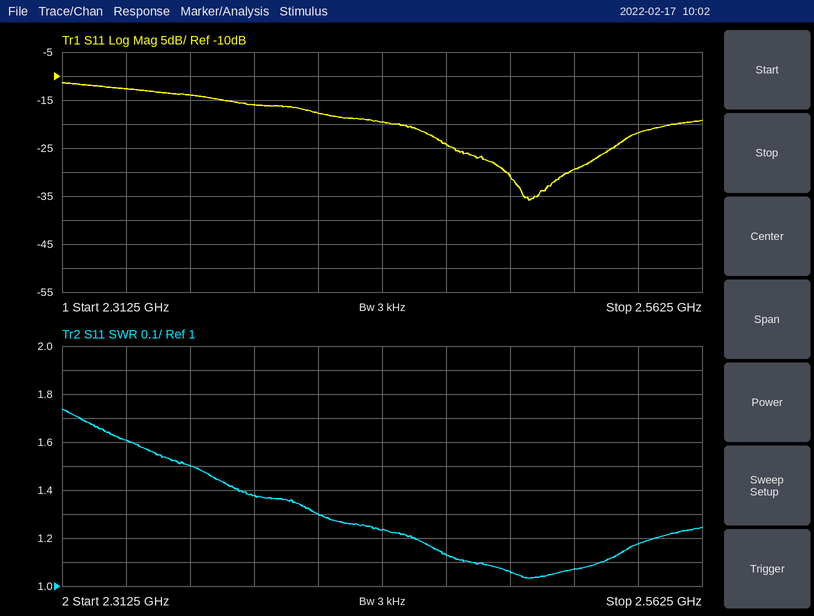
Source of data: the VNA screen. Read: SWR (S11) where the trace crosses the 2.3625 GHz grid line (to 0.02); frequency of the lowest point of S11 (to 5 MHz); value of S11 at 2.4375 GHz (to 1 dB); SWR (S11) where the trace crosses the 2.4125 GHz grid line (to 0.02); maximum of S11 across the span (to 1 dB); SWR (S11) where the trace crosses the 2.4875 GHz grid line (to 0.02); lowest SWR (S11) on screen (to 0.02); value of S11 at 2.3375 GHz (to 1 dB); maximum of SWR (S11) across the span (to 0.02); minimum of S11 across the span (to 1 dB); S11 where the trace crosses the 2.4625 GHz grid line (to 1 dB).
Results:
1.50
2.495 GHz
-20 dB
1.30
-11 dB
1.06
1.04
-13 dB
1.74
-36 dB
-24 dB
